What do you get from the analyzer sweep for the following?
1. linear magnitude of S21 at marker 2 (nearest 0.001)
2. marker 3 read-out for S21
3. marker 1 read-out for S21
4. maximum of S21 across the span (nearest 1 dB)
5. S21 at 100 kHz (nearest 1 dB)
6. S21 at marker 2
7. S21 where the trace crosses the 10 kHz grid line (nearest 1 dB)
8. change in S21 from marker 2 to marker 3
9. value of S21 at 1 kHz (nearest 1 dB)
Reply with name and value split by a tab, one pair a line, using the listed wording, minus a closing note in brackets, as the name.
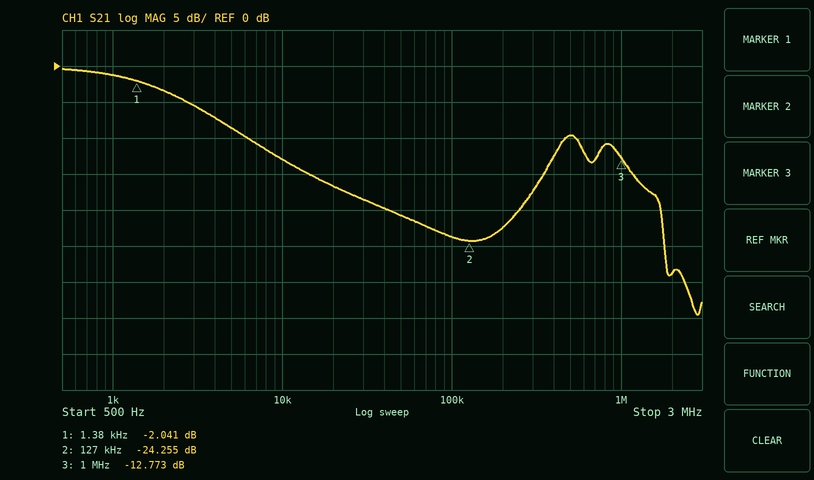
linear magnitude of S21 at marker 2	0.061
marker 3 read-out for S21	-12.773 dB
marker 1 read-out for S21	-2.041 dB
maximum of S21 across the span	0 dB
S21 at 100 kHz	-24 dB
S21 at marker 2	-24.255 dB
S21 where the trace crosses the 10 kHz grid line	-13 dB
change in S21 from marker 2 to marker 3	11.482 dB
value of S21 at 1 kHz	-1 dB
